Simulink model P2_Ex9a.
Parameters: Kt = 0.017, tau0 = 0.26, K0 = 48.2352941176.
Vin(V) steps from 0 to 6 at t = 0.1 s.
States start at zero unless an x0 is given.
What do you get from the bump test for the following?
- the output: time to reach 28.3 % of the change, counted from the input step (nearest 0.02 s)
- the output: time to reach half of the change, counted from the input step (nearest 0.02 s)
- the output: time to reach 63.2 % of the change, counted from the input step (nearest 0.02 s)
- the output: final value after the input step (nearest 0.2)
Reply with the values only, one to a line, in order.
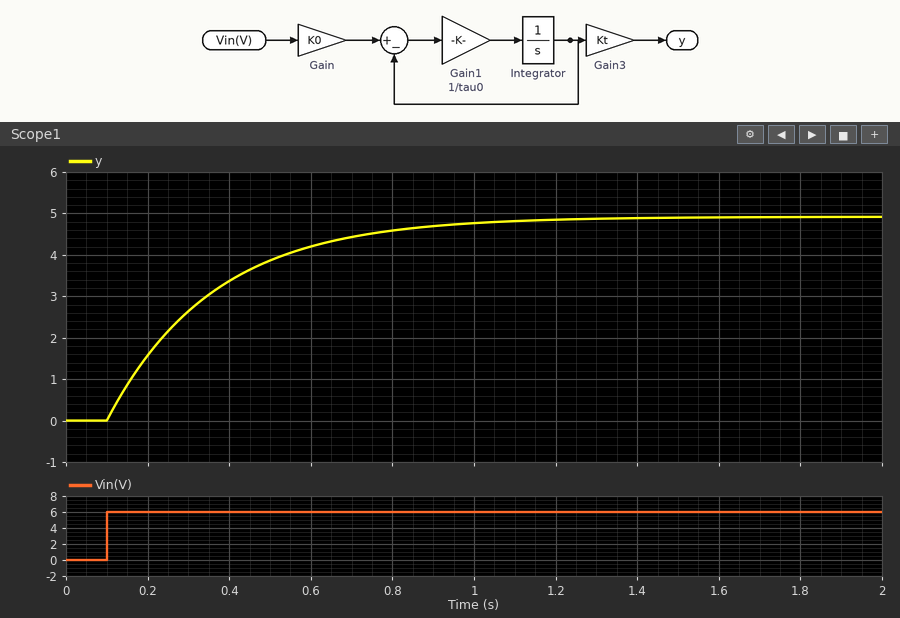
0.08 s
0.18 s
0.26 s
5.0
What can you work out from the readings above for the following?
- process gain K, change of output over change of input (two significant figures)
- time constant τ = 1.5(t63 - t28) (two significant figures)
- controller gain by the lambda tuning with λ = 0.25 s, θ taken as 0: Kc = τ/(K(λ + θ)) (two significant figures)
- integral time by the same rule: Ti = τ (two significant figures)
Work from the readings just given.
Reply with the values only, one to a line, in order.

0.83
0.27 s
1.3
0.27 s
